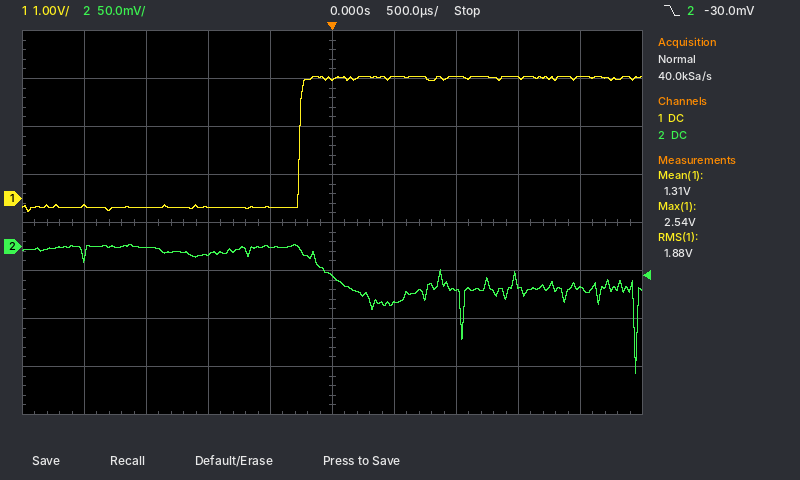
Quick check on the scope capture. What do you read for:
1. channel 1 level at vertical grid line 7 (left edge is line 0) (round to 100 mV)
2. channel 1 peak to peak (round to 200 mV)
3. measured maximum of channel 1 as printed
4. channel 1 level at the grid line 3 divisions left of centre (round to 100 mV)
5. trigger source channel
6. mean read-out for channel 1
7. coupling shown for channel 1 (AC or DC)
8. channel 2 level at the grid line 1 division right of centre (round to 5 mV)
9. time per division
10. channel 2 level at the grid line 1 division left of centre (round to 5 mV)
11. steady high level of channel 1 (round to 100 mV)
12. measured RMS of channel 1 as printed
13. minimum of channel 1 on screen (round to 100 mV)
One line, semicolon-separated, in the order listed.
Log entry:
2.5 V; 2.8 V; 2.54 V; -200 mV; channel 2; 1.31 V; DC; -60 mV; 500 µs; 0 mV; 2.5 V; 1.88 V; -300 mV
